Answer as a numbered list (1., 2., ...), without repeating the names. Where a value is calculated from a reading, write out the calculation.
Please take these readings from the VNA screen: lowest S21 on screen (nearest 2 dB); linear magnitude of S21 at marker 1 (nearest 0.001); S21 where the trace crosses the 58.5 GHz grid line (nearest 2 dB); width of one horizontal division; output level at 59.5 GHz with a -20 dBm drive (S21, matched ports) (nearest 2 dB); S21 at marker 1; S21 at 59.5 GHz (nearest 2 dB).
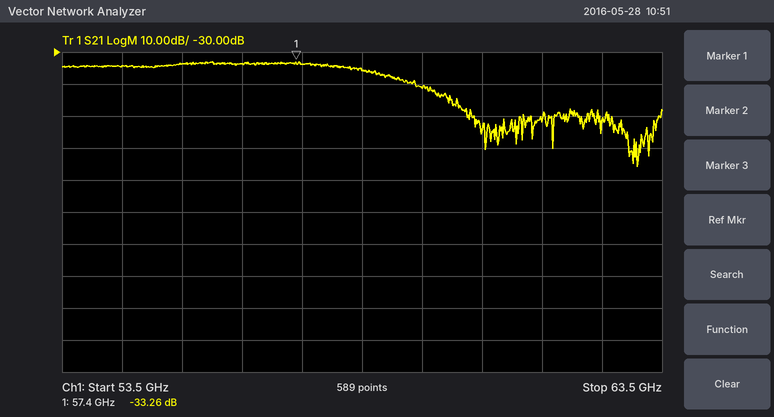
1. -66 dB
2. 10^(-33.26/20) ≈ 0.022
3. -36 dB
4. 1 GHz
5. -20 dBm + (-42 dB) = -62 dBm
6. -33.26 dB
7. -42 dB
